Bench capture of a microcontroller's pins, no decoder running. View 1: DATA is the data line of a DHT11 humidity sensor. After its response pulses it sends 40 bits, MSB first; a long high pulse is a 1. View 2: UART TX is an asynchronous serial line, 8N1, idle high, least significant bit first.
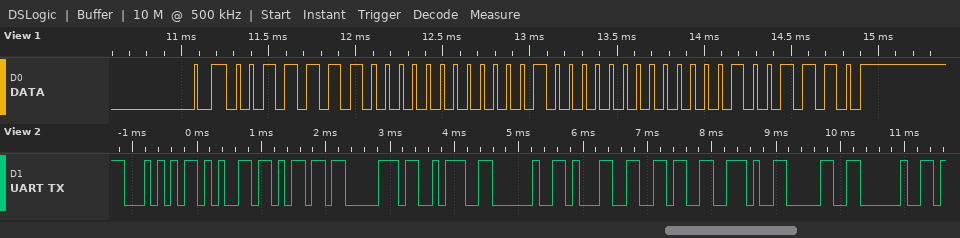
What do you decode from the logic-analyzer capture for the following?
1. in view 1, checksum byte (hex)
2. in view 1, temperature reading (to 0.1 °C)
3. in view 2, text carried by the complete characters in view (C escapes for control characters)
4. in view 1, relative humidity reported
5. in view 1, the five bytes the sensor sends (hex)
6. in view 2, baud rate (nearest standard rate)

0x4E
16.0 °C
"Temp: 16.0 "
62 %
3E 00 10 00 4E
9600 baud
